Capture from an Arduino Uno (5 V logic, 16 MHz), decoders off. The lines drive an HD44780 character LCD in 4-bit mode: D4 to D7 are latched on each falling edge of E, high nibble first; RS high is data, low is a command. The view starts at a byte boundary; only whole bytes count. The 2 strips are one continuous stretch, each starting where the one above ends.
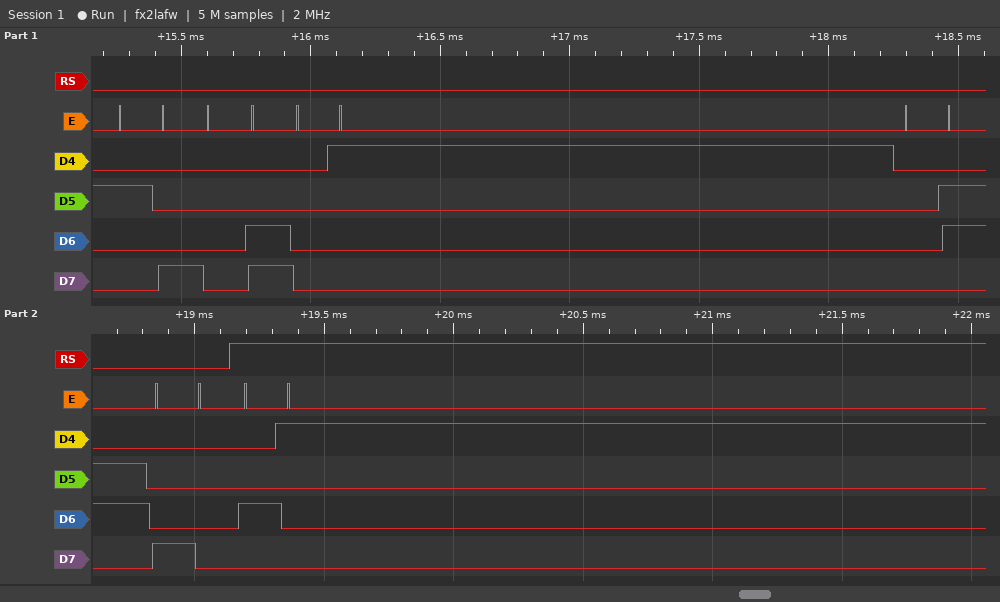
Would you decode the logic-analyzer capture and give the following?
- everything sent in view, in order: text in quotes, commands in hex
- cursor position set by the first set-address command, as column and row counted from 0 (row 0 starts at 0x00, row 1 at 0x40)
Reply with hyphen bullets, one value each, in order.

- 0x28 0x0C 0x01 0x06 0x80 "A"
- column 0, row 0
